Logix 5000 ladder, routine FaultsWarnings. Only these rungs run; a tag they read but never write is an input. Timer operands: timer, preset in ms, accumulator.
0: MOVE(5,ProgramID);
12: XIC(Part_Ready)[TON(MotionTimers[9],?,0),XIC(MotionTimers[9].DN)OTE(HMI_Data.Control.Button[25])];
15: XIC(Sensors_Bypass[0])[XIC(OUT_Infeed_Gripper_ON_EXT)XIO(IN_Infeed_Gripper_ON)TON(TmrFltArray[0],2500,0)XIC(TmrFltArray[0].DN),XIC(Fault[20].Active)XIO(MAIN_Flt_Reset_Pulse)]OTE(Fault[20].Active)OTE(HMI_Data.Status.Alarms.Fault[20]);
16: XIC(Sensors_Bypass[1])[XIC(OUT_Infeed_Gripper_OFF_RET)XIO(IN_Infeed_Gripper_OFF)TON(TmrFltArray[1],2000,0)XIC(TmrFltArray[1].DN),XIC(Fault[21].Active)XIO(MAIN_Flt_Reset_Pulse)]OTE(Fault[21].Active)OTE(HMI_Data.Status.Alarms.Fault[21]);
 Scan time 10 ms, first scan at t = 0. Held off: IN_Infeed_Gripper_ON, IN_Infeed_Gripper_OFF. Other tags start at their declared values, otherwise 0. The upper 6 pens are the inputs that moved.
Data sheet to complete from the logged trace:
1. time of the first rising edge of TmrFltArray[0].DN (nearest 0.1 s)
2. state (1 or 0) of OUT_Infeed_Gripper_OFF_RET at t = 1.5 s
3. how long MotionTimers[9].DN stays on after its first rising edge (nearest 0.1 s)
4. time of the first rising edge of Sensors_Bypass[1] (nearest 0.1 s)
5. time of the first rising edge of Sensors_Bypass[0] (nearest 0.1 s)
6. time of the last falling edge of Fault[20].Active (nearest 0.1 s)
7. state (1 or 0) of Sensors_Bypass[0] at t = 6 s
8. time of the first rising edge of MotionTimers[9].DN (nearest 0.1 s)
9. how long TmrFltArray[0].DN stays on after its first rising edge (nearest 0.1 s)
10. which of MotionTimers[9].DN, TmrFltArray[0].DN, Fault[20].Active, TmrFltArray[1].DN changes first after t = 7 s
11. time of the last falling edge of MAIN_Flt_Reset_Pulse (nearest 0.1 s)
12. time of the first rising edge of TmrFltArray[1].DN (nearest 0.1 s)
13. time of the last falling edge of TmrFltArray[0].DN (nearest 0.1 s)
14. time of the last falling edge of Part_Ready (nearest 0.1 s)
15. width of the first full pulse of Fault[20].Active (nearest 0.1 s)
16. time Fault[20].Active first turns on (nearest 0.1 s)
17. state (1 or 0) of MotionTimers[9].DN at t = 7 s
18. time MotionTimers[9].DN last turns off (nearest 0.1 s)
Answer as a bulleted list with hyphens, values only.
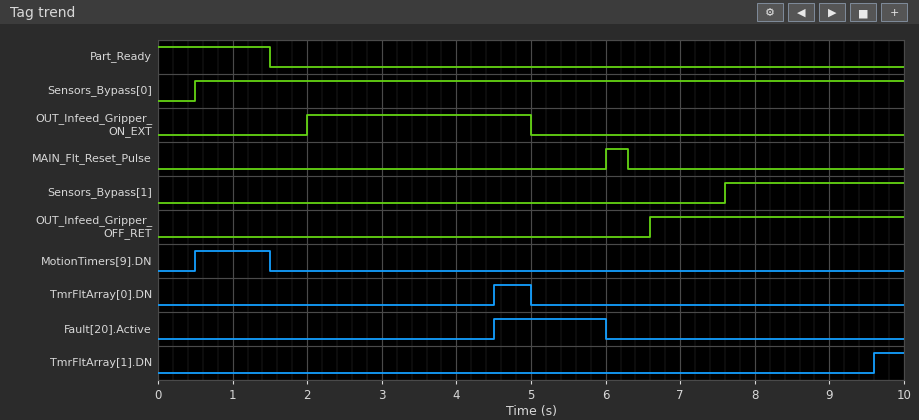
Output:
- 4.5 s
- 0
- 1.0 s
- 7.6 s
- 0.5 s
- 6.0 s
- 1
- 0.5 s
- 0.5 s
- TmrFltArray[1].DN
- 6.3 s
- 9.6 s
- 5.0 s
- 1.5 s
- 1.5 s
- 4.5 s
- 0
- 1.5 s
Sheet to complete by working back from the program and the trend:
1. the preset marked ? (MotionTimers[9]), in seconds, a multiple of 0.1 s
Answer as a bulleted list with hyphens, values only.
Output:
- 0.5 s
